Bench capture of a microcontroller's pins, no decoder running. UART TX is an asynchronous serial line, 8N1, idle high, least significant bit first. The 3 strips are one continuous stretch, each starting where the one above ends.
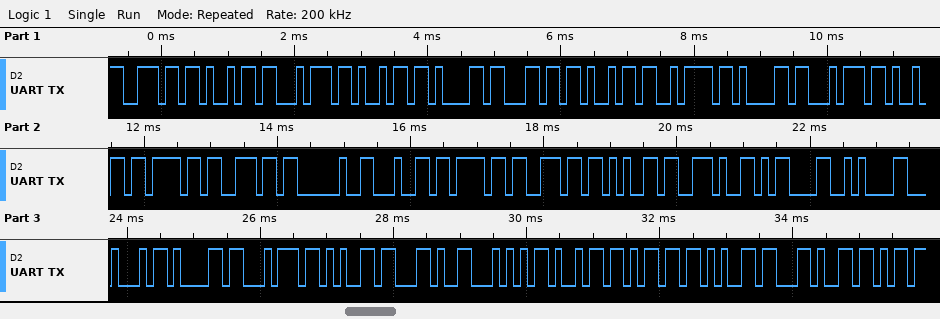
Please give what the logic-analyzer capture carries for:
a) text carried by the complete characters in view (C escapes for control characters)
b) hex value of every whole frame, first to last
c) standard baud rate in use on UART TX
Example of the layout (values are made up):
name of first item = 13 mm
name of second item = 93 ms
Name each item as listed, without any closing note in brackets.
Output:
text carried by the complete characters in view = "nitialization done.\r\nDate,Time,k"
hex value of every whole frame, first to last = 6E 69 74 69 61 6C 69 7A 61 74 69 6F 6E 20 64 6F 6E 65 2E 0D 0A 44 61 74 65 2C 54 69 6D 65 2C 6B
standard baud rate in use on UART TX = 9600 baud
